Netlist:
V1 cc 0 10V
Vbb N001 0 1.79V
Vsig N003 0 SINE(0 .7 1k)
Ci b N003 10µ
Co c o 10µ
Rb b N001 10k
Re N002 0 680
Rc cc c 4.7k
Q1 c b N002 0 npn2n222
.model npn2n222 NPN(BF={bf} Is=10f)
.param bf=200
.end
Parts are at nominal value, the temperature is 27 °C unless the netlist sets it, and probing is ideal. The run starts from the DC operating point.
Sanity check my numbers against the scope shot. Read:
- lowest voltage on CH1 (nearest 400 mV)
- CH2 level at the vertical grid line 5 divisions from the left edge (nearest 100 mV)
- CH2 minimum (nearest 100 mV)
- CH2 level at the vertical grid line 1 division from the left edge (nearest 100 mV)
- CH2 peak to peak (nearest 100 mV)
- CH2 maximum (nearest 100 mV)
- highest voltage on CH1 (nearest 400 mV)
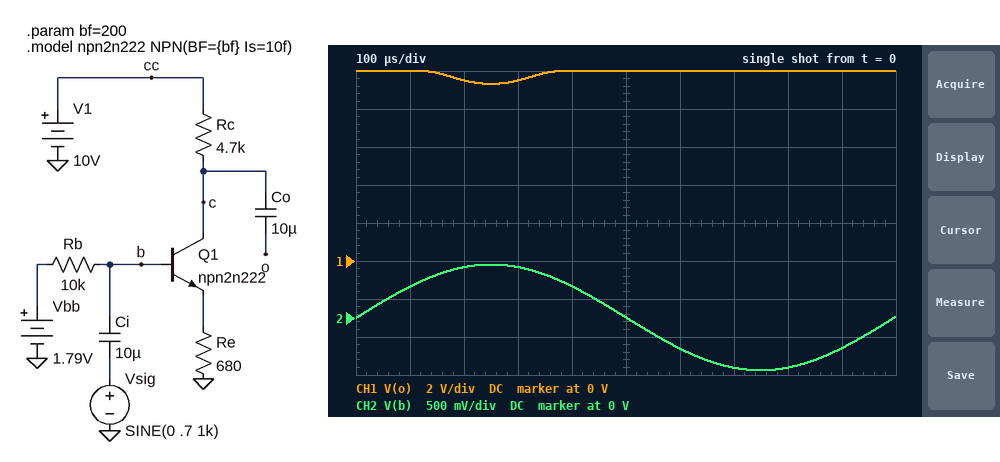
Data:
9.2 V
0 V
-700 mV
400 mV
1.4 V
700 mV
10.0 V
